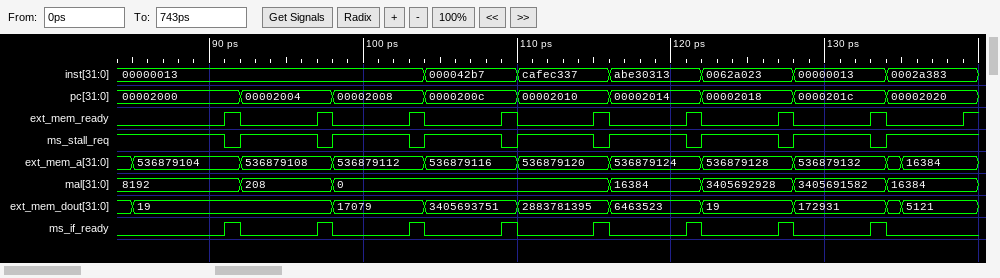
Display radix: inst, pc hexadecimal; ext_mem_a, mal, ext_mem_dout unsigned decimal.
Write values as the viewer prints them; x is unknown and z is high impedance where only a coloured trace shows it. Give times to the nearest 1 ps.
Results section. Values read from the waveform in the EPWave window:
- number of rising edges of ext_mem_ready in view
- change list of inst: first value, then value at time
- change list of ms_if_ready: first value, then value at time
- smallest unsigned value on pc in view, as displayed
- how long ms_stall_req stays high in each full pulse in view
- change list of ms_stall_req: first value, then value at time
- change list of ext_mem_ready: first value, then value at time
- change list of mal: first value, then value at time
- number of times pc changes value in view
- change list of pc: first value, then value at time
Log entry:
9
00000013, 000042b7 at 104 ps, cafec337 at 110 ps, abe30313 at 116 ps, 0062a023 at 122 ps, 00000013 at 128 ps, 0002a383 at 134 ps
0, 1 at 91 ps, 0 at 92 ps, 1 at 97 ps, 0 at 98 ps, 1 at 103 ps, 0 at 104 ps, 1 at 109 ps, 0 at 110 ps, 1 at 115 ps, 0 at 116 ps, 1 at 121 ps, 0 at 122 ps, 1 at 127 ps, 0 at 128 ps, 1 at 133 ps, 0 at 134 ps
00002000
5 ps, 5 ps, 5 ps, 5 ps, 5 ps, 5 ps, 5 ps
1, 0 at 91 ps, 1 at 92 ps, 0 at 97 ps, 1 at 98 ps, 0 at 103 ps, 1 at 104 ps, 0 at 109 ps, 1 at 110 ps, 0 at 115 ps, 1 at 116 ps, 0 at 121 ps, 1 at 122 ps, 0 at 127 ps, 1 at 128 ps, 0 at 133 ps, 1 at 134 ps
0, 1 at 91 ps, 0 at 92 ps, 1 at 97 ps, 0 at 98 ps, 1 at 103 ps, 0 at 104 ps, 1 at 109 ps, 0 at 110 ps, 1 at 115 ps, 0 at 116 ps, 1 at 121 ps, 0 at 122 ps, 1 at 127 ps, 0 at 128 ps, 1 at 133 ps, 0 at 134 ps, 1 at 139 ps
8192, 208 at 92 ps, 0 at 98 ps, 16384 at 116 ps, 3405692928 at 122 ps, 3405691582 at 128 ps, 16384 at 134 ps
8
00002000, 00002004 at 92 ps, 00002008 at 98 ps, 0000200c at 104 ps, 00002010 at 110 ps, 00002014 at 116 ps, 00002018 at 122 ps, 0000201c at 128 ps, 00002020 at 134 ps
